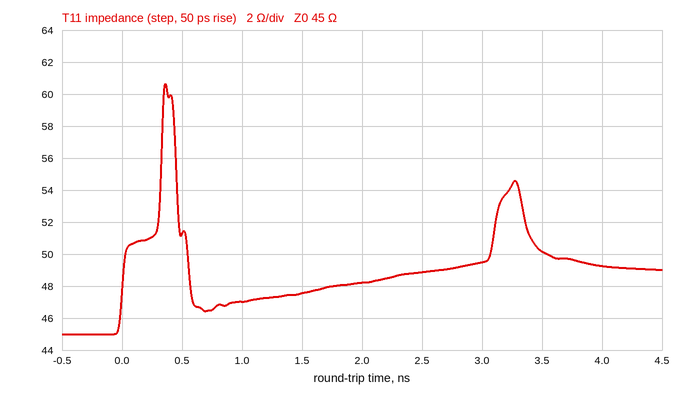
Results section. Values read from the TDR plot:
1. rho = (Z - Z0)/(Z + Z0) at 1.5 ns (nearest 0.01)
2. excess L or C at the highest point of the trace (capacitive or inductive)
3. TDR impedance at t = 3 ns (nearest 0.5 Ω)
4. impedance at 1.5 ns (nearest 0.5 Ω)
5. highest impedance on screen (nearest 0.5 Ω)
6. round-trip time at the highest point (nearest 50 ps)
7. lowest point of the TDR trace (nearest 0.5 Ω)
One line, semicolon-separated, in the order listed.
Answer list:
+0.03; inductive; 49.5 Ω; 47.5 Ω; 60.5 Ω; 350 ps; 45.0 Ω
